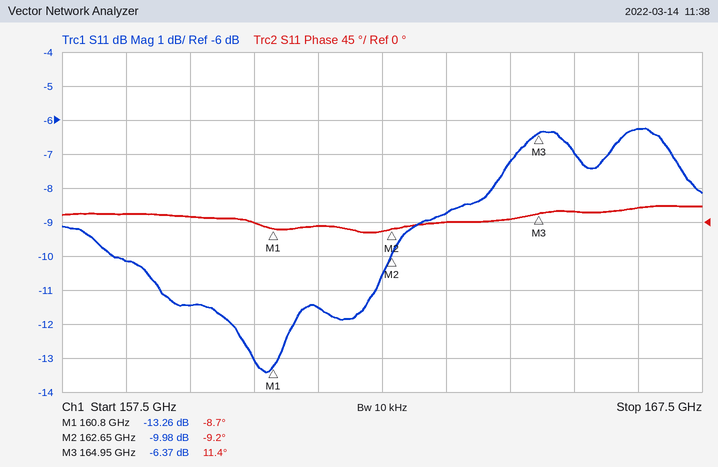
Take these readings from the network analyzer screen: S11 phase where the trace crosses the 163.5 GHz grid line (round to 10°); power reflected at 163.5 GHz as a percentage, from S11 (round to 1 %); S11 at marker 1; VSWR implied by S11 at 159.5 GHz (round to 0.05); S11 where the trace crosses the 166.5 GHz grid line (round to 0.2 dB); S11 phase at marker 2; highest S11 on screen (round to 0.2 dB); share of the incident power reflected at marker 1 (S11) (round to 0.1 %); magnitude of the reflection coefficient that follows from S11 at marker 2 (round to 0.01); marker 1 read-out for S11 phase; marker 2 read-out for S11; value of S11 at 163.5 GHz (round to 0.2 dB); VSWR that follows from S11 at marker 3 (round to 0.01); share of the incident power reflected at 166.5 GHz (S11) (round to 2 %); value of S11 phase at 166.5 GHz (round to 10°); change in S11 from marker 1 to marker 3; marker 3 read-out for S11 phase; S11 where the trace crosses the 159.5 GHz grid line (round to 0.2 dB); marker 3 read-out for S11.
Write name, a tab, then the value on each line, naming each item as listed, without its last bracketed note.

S11 phase where the trace crosses the 163.5 GHz grid line	0°
power reflected at 163.5 GHz as a percentage, from S11	13 %
S11 at marker 1	-13.26 dB
VSWR implied by S11 at 159.5 GHz	1.75
S11 where the trace crosses the 166.5 GHz grid line	-6.2 dB
S11 phase at marker 2	-9.2°
highest S11 on screen	-6.2 dB
share of the incident power reflected at marker 1 (S11)	4.7 %
magnitude of the reflection coefficient that follows from S11 at marker 2	0.32
marker 1 read-out for S11 phase	-8.7°
marker 2 read-out for S11	-9.98 dB
value of S11 at 163.5 GHz	-8.8 dB
VSWR that follows from S11 at marker 3	2.85
share of the incident power reflected at 166.5 GHz (S11)	24 %
value of S11 phase at 166.5 GHz	20°
change in S11 from marker 1 to marker 3	6.89 dB
marker 3 read-out for S11 phase	11.4°
S11 where the trace crosses the 159.5 GHz grid line	-11.4 dB
marker 3 read-out for S11	-6.37 dB
